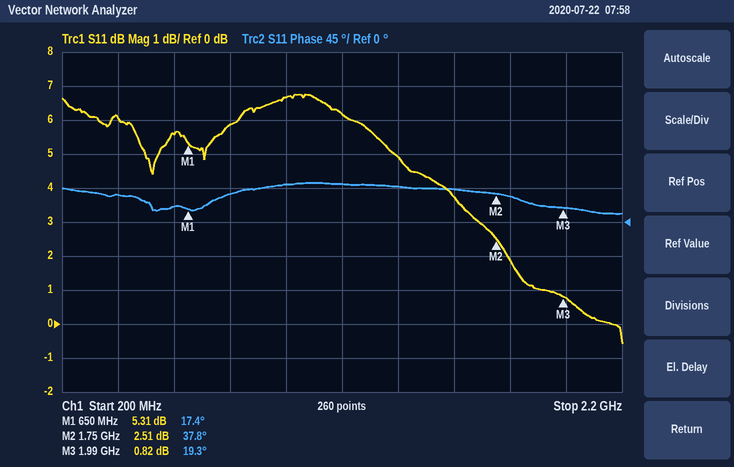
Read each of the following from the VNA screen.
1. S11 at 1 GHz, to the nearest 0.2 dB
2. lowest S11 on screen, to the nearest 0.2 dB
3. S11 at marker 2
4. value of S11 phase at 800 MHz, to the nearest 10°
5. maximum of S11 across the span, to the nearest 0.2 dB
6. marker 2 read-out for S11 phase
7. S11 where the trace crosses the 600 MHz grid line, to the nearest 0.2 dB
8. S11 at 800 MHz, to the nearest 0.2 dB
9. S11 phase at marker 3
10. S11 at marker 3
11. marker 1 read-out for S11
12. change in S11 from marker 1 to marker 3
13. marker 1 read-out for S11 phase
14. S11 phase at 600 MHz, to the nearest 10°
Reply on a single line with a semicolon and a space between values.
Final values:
6.6 dB; -0.6 dB; 2.51 dB; 40°; 6.8 dB; 37.8°; 5.6 dB; 5.8 dB; 19.3°; 0.82 dB; 5.31 dB; -4.49 dB; 17.4°; 20°
